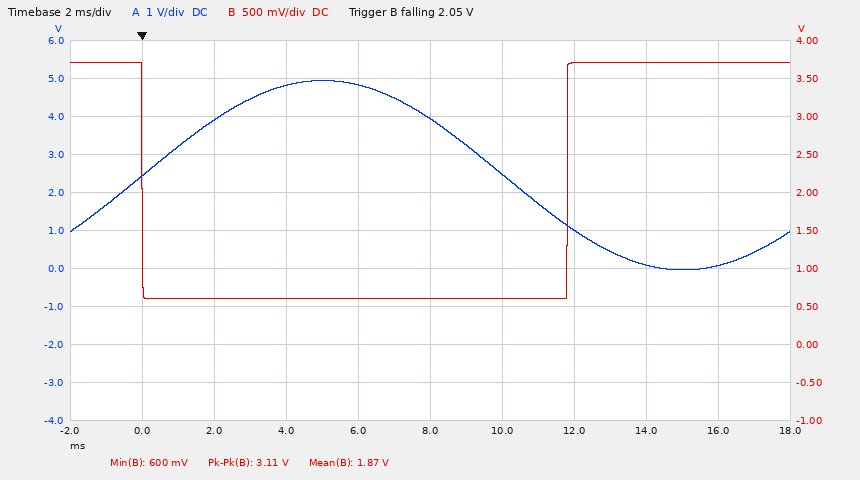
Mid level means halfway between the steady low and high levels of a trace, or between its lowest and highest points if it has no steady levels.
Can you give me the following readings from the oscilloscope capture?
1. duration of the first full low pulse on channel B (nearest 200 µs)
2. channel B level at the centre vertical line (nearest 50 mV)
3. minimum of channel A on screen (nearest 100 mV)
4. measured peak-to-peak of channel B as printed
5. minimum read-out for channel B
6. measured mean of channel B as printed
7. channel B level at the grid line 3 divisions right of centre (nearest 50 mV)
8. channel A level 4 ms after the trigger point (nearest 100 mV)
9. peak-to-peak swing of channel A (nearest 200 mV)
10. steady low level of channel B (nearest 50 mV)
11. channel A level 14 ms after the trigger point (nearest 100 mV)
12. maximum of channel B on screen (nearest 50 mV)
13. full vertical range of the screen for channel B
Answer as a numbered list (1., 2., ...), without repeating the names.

1. 11.8 ms
2. 600 mV
3. 0.0 V
4. 3.11 V
5. 600 mV
6. 1.87 V
7. 3.70 V
8. 4.8 V
9. 5.0 V
10. 600 mV
11. 100 mV
12. 3.70 V
13. 5 V
